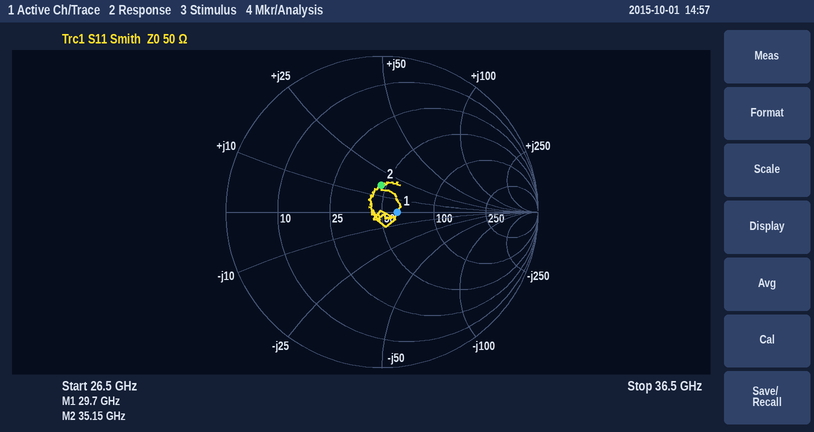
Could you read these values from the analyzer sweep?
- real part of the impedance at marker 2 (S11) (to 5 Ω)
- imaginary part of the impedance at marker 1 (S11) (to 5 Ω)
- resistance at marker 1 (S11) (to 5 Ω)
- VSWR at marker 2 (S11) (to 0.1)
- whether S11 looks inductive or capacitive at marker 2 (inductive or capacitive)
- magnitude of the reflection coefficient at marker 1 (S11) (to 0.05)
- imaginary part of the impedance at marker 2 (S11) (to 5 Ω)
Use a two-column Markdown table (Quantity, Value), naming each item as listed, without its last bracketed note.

| Quantity | Value |
|---|---|
| real part of the impedance at marker 2 (S11) | 45 Ω |
| imaginary part of the impedance at marker 1 (S11) | 0 Ω |
| resistance at marker 1 (S11) | 60 Ω |
| VSWR at marker 2 (S11) | 1.4 |
| whether S11 looks inductive or capacitive at marker 2 | inductive |
| magnitude of the reflection coefficient at marker 1 (S11) | 0.10 |
| imaginary part of the impedance at marker 2 (S11) | +15 Ω |
